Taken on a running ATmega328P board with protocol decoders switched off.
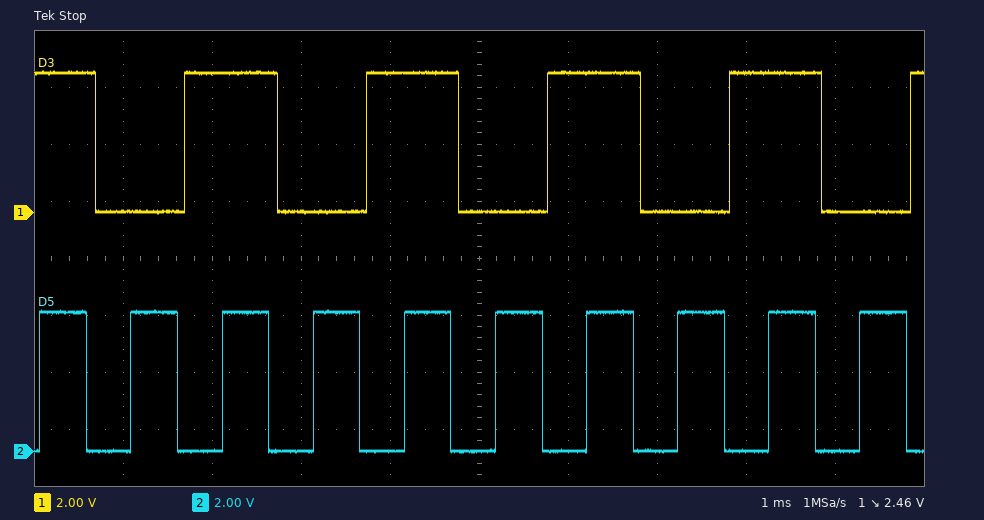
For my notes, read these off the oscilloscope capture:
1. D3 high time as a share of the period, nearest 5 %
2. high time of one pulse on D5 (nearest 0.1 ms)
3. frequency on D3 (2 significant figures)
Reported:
50 %
0.5 ms
490 Hz
